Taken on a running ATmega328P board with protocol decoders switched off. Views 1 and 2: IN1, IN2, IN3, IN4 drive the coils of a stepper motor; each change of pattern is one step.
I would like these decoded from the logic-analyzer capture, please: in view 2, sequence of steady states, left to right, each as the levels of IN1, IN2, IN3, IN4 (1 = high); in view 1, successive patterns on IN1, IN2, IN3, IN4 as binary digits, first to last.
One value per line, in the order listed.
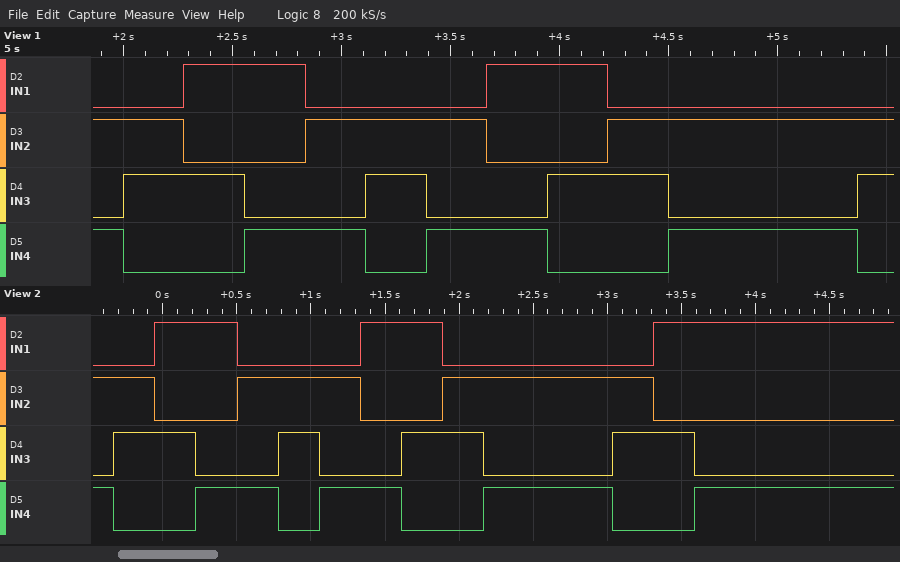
0101 0110 1010 1001 0101 0110 0101 1001 1010 0110 0101 0110 1010 1001
0101 0110 1010 1001 0101 0110 0101 1001 1010 0110 0101 0110
